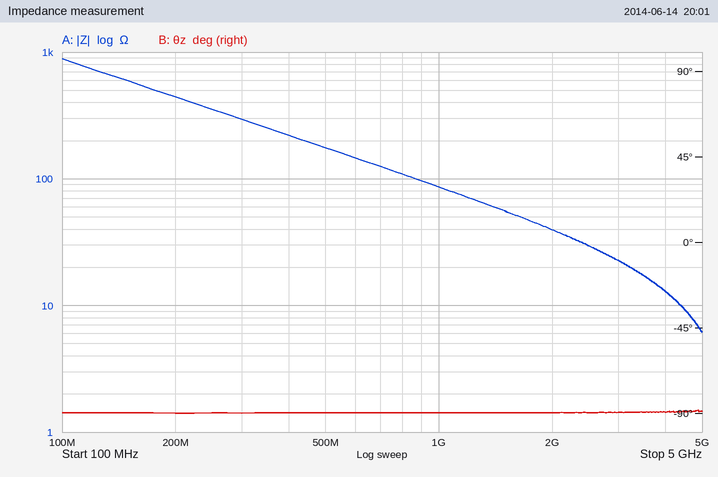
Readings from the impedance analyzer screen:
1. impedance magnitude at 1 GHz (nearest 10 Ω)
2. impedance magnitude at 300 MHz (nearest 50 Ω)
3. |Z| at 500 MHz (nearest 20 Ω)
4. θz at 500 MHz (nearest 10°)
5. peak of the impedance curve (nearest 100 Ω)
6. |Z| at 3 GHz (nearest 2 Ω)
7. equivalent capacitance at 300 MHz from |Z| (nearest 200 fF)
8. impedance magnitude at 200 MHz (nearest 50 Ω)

90 Ω
300 Ω
180 Ω
-90°
900 Ω
22 Ω
1.8 pF
450 Ω
